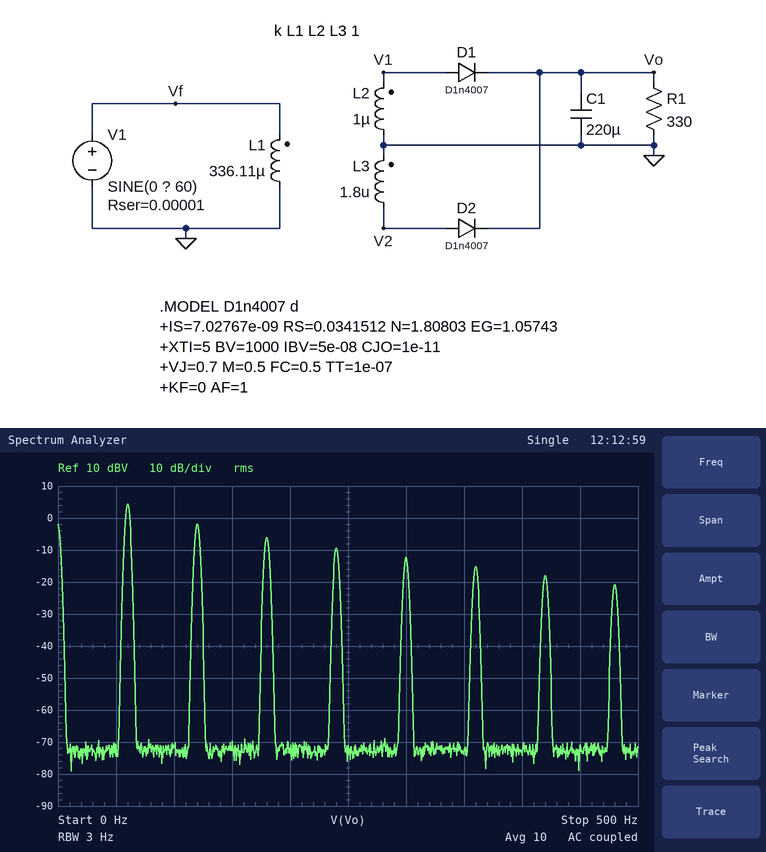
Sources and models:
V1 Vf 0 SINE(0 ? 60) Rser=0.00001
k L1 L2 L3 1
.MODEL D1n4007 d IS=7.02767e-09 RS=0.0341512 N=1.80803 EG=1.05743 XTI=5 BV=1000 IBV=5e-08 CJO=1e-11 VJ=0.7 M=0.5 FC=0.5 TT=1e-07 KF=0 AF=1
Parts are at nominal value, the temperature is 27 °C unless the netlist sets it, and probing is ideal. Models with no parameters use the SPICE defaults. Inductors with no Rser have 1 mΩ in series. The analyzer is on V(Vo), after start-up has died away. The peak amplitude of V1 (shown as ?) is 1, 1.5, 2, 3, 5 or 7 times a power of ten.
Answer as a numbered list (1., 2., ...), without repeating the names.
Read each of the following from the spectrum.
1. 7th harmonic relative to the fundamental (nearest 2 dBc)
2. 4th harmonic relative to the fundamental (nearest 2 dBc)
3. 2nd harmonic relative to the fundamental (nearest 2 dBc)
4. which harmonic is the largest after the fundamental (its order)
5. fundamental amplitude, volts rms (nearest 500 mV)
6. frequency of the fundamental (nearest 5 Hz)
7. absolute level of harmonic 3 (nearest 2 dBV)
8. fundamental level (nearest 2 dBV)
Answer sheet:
1. -22 dBc
2. -14 dBc
3. -6 dBc
4. 2
5. 1.5 V
6. 60 Hz
7. -6 dBV
8. 4 dBV
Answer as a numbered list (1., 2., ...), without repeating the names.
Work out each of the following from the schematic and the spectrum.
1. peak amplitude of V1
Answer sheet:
1. 500 V
